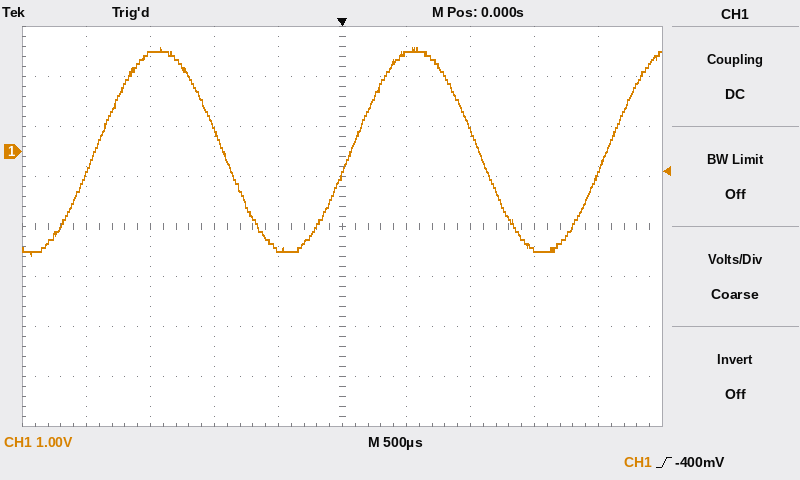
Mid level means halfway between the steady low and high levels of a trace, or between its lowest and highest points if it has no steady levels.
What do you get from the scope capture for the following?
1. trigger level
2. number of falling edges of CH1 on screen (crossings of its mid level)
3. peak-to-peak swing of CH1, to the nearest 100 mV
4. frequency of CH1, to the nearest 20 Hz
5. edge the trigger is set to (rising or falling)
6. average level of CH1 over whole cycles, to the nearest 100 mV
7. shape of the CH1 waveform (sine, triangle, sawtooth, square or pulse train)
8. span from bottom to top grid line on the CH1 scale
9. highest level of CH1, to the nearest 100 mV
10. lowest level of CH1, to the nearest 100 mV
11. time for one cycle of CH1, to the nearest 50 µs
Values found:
-400 mV
2
4.2 V
500 Hz
rising
0.0 V
sine
8 V
2.1 V
-2.1 V
2.00 ms
